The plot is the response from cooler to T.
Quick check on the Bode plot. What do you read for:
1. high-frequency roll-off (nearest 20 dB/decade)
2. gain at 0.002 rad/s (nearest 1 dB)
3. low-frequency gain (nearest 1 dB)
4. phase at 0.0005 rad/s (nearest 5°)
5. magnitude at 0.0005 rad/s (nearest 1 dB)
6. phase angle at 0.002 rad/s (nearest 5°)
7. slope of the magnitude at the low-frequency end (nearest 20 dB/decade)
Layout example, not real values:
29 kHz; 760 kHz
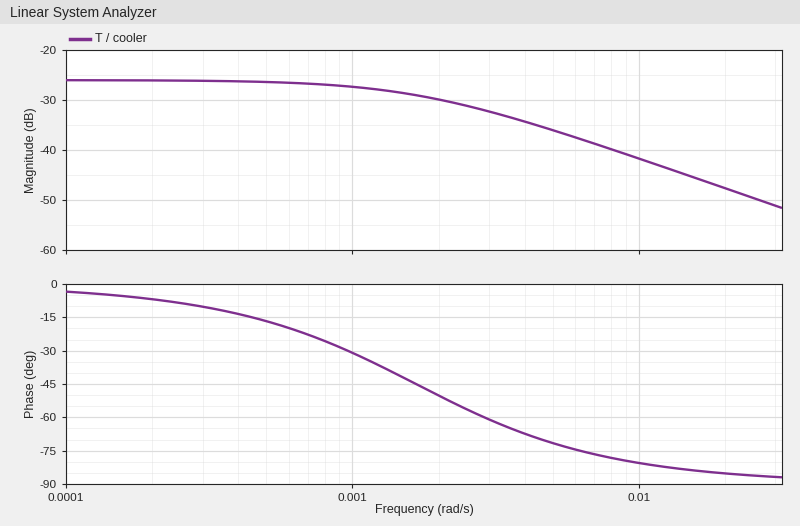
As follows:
-20 dB/decade; -30 dB; -26 dB; -15°; -26 dB; -50°; 0 dB/decade
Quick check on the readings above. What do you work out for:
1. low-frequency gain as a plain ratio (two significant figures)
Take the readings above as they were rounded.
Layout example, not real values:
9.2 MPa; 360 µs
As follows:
0.050
